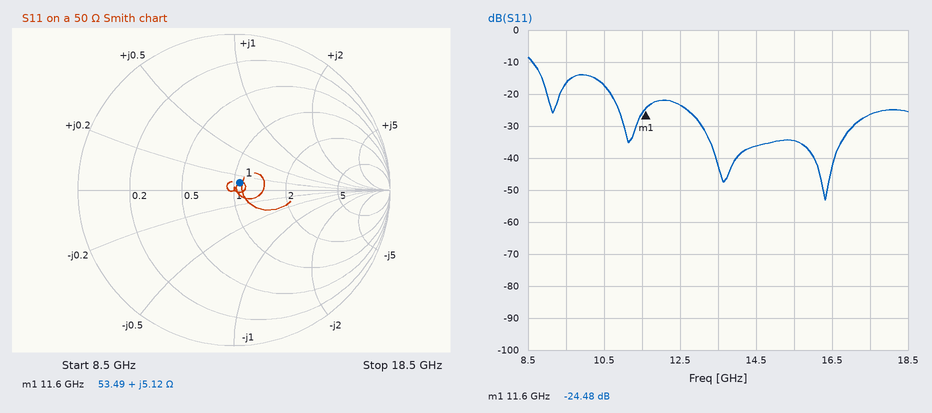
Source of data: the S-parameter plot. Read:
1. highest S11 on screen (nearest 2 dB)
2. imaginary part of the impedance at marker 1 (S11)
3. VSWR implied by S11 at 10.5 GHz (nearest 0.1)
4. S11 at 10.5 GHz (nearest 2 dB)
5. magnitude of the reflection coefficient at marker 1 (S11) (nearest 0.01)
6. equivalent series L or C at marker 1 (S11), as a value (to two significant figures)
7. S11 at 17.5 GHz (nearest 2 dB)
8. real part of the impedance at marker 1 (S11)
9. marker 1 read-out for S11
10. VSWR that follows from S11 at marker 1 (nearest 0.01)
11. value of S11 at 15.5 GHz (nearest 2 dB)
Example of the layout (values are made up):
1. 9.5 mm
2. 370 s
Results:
1. -8 dB
2. +5.12 Ω
3. 1.3
4. -18 dB
5. 0.06
6. 70 pH
7. -26 dB
8. 53.49 Ω
9. -24.48 dB
10. 1.13
11. -34 dB
